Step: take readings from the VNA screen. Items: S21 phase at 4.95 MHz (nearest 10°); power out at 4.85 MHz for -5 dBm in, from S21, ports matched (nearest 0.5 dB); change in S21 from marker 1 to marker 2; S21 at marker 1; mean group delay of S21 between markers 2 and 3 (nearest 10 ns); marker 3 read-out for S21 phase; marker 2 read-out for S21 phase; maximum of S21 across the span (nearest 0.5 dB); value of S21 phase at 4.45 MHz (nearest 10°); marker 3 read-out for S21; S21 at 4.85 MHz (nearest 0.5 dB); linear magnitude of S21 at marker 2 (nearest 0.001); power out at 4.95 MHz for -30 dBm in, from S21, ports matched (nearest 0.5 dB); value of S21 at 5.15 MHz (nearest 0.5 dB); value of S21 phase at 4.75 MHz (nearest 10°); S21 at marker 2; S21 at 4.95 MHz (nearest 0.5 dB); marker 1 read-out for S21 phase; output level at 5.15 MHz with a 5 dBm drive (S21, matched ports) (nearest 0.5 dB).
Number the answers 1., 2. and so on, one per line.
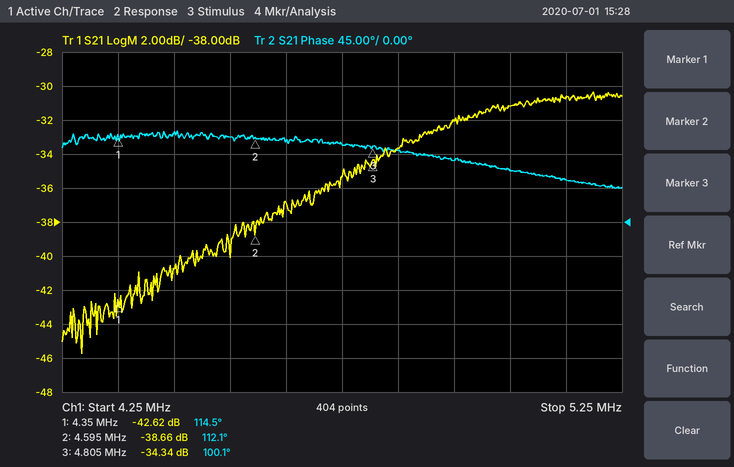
1. 80°
2. -38.5 dBm
3. 3.96 dB
4. -42.62 dB
5. 160 ns
6. 100.1°
7. 112.1°
8. -30.5 dB
9. 120°
10. -34.34 dB
11. -33.5 dB
12. 0.012
13. -62.0 dBm
14. -30.5 dB
15. 100°
16. -38.66 dB
17. -32.0 dB
18. 114.5°
19. -25.5 dBm
